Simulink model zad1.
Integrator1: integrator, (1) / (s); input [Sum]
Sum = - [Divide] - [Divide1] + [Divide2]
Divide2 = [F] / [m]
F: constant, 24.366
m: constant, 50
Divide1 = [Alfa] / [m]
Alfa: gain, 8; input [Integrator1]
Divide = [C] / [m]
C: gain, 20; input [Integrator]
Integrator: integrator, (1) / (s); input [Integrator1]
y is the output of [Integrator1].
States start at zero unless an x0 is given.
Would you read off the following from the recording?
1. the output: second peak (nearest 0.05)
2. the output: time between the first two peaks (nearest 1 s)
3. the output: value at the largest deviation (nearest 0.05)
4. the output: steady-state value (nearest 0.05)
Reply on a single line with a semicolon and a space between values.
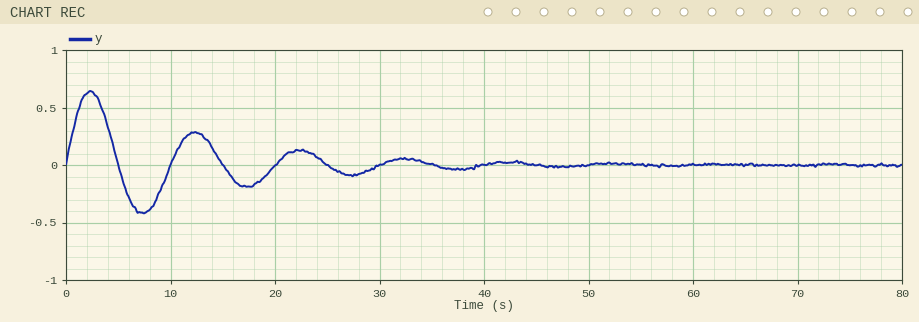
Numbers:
0.30; 10 s; 0.65; 0.00
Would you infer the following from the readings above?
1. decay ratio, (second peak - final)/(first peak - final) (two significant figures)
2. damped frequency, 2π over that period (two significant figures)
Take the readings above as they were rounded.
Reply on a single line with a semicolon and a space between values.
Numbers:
0.46; 0.63 rad/s
